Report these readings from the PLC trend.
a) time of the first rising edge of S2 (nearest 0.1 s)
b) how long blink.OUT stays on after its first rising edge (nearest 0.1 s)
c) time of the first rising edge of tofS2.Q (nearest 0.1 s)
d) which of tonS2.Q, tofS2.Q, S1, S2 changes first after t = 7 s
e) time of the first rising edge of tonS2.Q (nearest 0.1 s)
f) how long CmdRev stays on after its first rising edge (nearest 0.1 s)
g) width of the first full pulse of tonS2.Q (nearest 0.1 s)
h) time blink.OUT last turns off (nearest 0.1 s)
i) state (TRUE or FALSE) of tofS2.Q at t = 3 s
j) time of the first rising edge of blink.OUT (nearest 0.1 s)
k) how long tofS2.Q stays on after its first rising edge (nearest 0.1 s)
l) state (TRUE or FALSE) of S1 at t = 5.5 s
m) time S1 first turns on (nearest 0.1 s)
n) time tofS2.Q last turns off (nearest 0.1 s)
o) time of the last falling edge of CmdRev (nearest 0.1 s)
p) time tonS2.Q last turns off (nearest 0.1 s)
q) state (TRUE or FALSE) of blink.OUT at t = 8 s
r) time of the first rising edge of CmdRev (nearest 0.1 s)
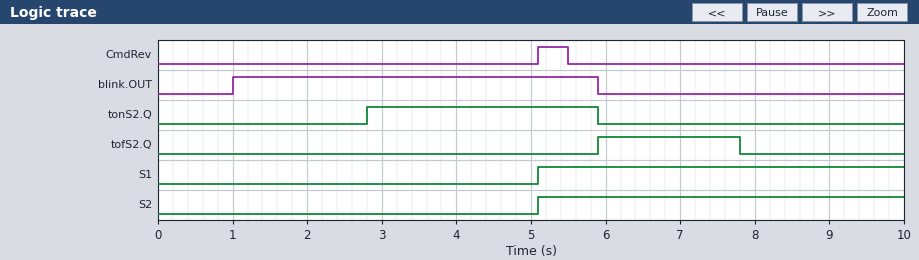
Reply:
5.1 s
4.9 s
5.9 s
tofS2.Q
2.8 s
0.4 s
3.1 s
5.9 s
FALSE
1.0 s
1.9 s
TRUE
5.1 s
7.8 s
5.5 s
5.9 s
FALSE
5.1 s
